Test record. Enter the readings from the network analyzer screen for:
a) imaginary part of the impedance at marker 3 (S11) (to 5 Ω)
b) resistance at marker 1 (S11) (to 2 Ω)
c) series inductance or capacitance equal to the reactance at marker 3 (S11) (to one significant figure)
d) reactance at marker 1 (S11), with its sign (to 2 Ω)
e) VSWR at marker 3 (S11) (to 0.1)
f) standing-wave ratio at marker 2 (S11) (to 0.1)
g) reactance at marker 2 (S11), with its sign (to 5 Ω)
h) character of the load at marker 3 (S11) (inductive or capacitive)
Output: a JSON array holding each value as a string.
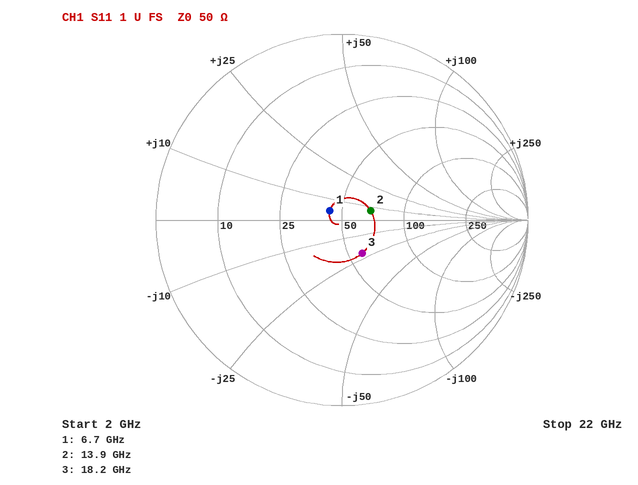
["-20 Ω", "44 Ω", "400 fF", "+4 Ω", "1.5", "1.4", "+5 Ω", "capacitive"]
